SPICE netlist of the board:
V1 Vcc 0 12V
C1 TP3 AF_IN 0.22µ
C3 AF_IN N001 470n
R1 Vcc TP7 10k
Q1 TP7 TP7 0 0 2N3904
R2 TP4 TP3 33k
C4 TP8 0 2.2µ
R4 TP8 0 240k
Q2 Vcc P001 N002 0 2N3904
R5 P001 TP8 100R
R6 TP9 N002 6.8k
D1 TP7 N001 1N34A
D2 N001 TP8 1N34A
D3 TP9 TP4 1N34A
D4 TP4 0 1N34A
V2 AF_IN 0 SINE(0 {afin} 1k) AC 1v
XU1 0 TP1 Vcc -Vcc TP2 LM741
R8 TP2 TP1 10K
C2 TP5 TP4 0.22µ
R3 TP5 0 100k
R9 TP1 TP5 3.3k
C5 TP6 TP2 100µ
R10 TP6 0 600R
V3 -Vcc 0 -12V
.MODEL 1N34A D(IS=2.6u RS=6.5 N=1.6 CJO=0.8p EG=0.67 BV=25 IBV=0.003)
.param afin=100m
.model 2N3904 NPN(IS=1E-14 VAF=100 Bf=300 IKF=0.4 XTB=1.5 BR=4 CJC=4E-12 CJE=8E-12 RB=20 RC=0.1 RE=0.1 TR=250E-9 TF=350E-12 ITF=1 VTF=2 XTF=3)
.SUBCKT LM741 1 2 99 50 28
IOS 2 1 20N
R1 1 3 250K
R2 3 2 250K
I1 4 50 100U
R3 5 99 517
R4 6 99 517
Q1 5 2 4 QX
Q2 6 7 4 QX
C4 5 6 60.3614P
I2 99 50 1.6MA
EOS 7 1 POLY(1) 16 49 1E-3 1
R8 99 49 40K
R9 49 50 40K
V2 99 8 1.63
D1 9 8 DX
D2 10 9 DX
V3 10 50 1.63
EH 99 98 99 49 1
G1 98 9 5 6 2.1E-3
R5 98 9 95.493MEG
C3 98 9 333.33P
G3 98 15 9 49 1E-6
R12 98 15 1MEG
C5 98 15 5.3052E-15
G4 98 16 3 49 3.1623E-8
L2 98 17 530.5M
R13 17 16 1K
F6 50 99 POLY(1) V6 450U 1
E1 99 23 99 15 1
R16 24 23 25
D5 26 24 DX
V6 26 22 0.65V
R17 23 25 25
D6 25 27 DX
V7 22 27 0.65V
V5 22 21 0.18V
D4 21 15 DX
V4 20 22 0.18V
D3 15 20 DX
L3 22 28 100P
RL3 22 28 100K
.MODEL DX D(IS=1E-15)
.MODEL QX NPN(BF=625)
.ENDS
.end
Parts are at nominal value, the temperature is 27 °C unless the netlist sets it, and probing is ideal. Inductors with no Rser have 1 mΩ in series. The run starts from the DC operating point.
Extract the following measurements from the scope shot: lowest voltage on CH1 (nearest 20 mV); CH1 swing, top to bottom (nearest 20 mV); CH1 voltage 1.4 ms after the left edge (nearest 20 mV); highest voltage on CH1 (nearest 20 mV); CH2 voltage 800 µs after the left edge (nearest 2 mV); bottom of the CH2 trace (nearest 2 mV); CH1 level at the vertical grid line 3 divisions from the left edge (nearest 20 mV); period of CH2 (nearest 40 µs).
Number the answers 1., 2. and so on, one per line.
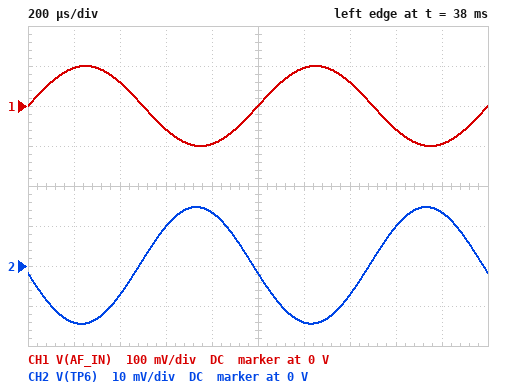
1. -100 mV
2. 200 mV
3. 60 mV
4. 100 mV
5. 14 mV
6. -14 mV
7. -60 mV
8. 1.00 ms
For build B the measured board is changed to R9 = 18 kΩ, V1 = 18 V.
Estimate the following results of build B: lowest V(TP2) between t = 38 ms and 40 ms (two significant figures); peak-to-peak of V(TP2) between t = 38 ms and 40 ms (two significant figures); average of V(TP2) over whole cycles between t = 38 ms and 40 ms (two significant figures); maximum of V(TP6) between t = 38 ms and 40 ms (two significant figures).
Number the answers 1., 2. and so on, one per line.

1. -2.5 mV
2. 8.5 mV
3. 1.7 mV
4. 4.3 mV
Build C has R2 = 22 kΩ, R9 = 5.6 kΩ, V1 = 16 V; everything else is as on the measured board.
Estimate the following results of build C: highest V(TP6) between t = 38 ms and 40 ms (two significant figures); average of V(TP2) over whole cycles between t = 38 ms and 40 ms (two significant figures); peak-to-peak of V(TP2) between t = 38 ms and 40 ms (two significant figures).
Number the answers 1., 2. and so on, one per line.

1. 16 mV
2. 1.7 mV
3. 31 mV
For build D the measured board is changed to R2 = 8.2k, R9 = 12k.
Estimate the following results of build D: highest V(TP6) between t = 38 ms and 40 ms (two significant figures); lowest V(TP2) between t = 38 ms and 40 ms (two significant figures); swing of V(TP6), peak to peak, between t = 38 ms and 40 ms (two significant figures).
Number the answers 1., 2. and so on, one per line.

1. 22 mV
2. -18 mV
3. 41 mV
